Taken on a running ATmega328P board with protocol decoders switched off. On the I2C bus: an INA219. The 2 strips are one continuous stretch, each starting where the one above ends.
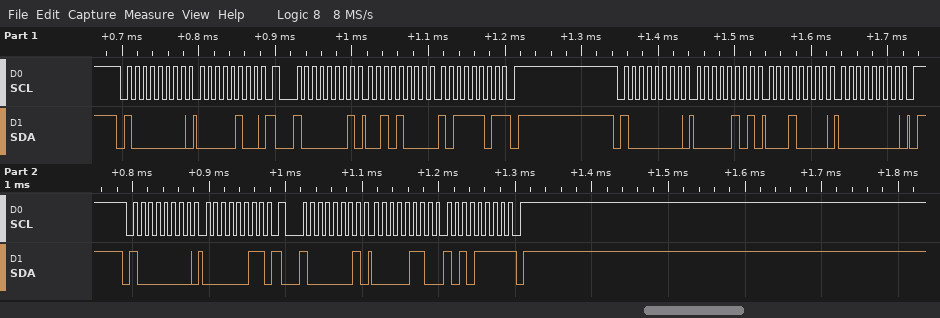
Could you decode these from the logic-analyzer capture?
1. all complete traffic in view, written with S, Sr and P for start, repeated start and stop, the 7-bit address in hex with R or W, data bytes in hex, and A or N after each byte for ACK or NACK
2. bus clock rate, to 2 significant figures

S 40W A 04 A Sr 40R A 28 A BD N P S 40W A 05 A 10 A 00 A P S 40W A 03 A Sr 40R A 06 A AF N P
100 kHz
